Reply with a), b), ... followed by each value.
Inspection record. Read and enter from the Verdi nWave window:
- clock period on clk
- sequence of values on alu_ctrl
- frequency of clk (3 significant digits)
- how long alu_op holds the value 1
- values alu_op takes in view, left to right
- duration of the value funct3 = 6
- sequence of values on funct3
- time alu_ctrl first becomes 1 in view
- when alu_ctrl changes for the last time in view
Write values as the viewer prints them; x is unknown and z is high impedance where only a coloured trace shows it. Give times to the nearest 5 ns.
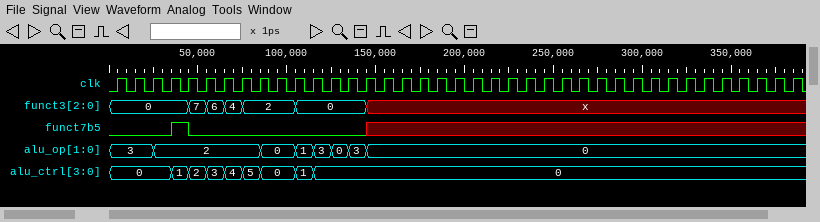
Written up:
a) 10 ns
b) 0, 1, 2, 3, 4, 5, 0, 1, 0
c) 100 MHz
d) 10 ns
e) 3, 2, 0, 1, 3, 0, 3, 0
f) 10 ns
g) 0, 7, 6, 4, 2, 0, x
h) 35 ns
i) 115 ns
